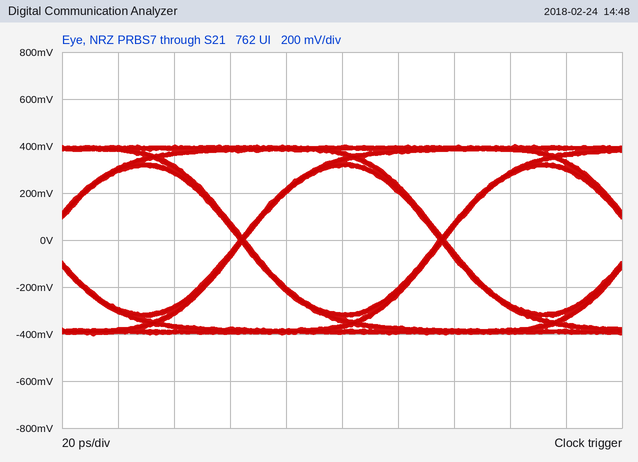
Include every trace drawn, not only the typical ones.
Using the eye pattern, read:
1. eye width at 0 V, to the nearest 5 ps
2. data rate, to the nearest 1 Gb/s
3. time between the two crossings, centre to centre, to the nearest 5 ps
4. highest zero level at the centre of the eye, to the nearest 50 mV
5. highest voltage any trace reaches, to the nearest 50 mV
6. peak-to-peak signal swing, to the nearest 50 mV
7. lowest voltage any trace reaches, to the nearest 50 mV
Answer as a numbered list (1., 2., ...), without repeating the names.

1. 70 ps
2. 14 Gb/s
3. 70 ps
4. -300 mV
5. 400 mV
6. 800 mV
7. -400 mV
